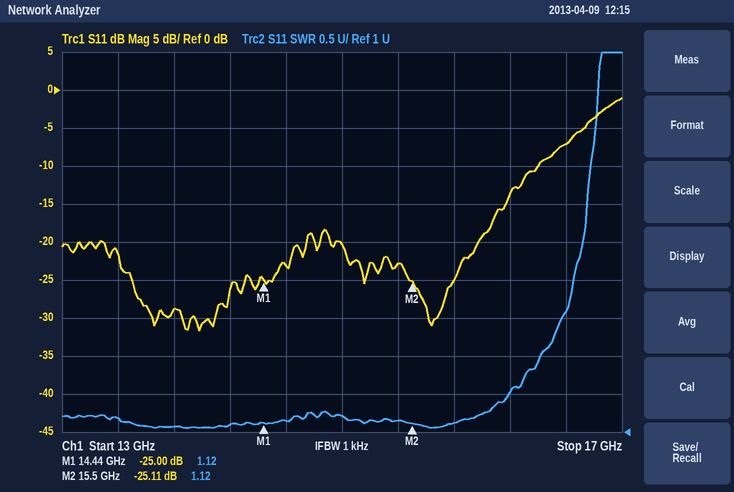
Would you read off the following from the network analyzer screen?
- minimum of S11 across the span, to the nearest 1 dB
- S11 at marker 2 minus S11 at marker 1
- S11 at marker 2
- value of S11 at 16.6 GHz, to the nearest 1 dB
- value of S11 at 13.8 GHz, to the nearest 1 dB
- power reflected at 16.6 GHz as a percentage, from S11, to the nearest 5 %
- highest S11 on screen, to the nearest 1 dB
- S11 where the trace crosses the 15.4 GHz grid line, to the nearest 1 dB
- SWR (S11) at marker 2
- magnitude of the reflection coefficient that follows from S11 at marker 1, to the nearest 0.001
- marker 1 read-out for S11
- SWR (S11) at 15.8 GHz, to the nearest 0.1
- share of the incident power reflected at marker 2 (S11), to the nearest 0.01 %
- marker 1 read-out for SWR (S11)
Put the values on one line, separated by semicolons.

-32 dB; -0.11 dB; -25.11 dB; -7 dB; -29 dB; 20 %; -1 dB; -23 dB; 1.12; 0.056; -25.00 dB; 1.1; 0.31 %; 1.12
